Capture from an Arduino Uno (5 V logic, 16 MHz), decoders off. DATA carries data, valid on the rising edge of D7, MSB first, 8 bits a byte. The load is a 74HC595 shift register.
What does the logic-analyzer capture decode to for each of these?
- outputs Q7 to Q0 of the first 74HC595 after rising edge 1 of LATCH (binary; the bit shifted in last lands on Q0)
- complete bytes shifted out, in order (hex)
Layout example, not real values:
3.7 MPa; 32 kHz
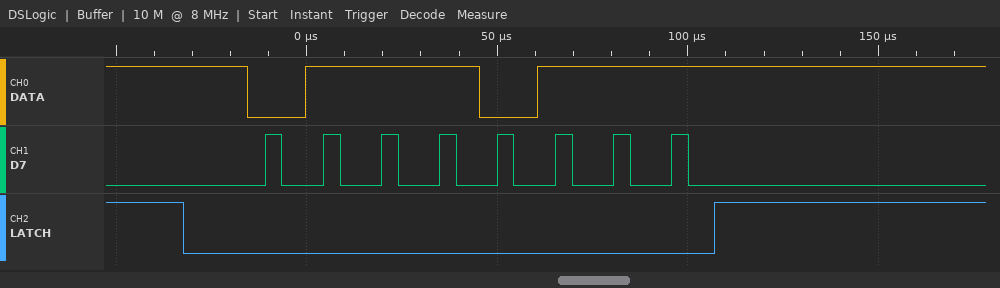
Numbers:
01110111; 0x77
